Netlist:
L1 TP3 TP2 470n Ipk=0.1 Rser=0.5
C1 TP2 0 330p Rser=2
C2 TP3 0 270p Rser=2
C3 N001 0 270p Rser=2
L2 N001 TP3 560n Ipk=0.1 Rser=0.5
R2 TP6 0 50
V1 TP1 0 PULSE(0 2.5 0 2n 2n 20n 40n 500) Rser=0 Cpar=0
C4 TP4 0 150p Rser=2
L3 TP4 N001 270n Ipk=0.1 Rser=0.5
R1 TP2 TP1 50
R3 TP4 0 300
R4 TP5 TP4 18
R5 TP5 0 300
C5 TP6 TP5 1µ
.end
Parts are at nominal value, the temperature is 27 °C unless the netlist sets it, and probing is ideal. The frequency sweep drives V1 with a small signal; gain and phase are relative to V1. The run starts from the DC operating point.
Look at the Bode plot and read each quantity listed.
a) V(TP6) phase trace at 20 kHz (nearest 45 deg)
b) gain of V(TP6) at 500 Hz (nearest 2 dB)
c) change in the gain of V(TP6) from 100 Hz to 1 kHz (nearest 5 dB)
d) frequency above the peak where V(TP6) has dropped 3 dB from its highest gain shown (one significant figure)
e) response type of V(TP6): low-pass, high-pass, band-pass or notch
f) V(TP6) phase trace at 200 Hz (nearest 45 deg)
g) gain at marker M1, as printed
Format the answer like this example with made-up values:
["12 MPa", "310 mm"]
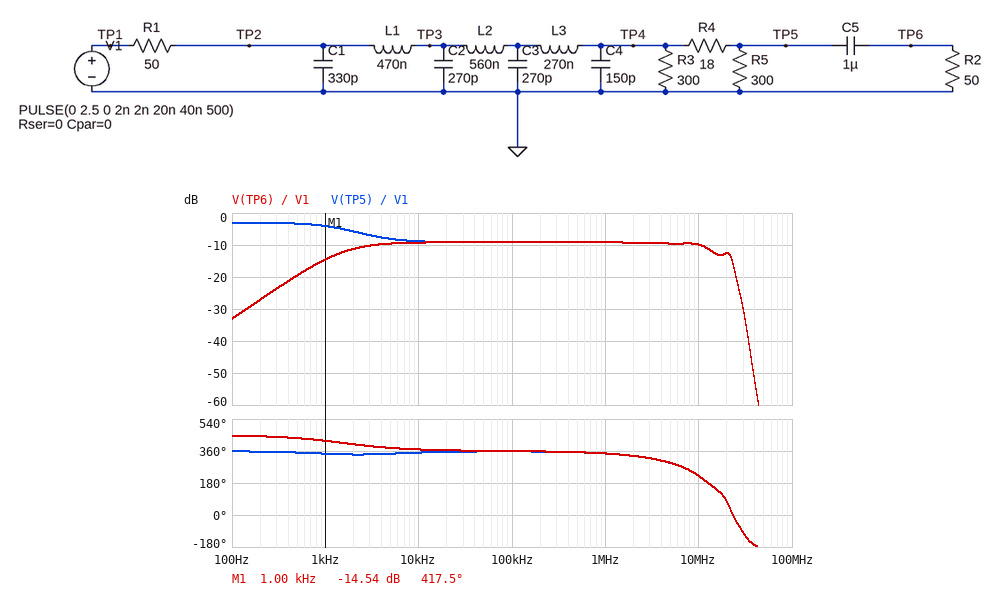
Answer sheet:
["360 deg", "-20 dB", "20 dB", "10 MHz", "band-pass", "450 deg", "-14.54 dB"]
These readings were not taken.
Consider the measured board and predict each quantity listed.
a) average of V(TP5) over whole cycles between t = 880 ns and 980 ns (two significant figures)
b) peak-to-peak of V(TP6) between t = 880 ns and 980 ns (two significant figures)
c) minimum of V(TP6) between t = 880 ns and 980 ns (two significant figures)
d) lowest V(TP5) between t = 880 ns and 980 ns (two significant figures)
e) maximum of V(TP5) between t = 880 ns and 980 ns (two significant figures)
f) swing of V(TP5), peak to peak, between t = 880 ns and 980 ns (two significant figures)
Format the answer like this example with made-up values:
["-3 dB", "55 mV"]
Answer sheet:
["480 mV", "330 mV", "310 mV", "320 mV", "650 mV", "330 mV"]
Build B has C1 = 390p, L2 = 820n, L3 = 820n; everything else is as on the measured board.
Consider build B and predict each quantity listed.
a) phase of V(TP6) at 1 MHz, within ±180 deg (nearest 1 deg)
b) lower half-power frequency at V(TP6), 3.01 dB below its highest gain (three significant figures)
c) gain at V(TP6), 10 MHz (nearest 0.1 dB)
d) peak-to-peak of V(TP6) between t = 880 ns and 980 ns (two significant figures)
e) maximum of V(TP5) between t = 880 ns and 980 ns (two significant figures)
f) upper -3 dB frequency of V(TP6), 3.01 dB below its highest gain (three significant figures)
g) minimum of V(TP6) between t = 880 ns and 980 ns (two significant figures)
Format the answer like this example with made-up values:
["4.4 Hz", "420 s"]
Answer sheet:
["-17 deg", "1.57 kHz", "-11.3 dB", "59 mV", "510 mV", "15.4 MHz", "450 mV"]
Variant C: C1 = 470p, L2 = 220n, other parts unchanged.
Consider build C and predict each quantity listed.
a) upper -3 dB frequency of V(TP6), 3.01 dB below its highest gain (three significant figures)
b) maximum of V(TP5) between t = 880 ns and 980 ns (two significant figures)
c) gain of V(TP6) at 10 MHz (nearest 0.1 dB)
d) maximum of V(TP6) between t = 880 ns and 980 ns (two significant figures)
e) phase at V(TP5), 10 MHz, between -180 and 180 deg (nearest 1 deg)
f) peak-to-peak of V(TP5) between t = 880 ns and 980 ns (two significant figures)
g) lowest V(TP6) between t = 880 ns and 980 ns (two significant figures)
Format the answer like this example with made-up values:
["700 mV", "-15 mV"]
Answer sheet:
["14.4 MHz", "630 mV", "-10.0 dB", "620 mV", "-126 deg", "300 mV", "330 mV"]
